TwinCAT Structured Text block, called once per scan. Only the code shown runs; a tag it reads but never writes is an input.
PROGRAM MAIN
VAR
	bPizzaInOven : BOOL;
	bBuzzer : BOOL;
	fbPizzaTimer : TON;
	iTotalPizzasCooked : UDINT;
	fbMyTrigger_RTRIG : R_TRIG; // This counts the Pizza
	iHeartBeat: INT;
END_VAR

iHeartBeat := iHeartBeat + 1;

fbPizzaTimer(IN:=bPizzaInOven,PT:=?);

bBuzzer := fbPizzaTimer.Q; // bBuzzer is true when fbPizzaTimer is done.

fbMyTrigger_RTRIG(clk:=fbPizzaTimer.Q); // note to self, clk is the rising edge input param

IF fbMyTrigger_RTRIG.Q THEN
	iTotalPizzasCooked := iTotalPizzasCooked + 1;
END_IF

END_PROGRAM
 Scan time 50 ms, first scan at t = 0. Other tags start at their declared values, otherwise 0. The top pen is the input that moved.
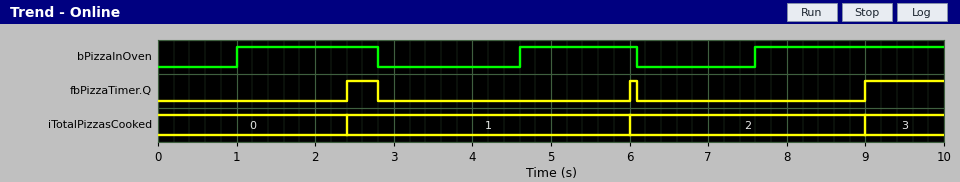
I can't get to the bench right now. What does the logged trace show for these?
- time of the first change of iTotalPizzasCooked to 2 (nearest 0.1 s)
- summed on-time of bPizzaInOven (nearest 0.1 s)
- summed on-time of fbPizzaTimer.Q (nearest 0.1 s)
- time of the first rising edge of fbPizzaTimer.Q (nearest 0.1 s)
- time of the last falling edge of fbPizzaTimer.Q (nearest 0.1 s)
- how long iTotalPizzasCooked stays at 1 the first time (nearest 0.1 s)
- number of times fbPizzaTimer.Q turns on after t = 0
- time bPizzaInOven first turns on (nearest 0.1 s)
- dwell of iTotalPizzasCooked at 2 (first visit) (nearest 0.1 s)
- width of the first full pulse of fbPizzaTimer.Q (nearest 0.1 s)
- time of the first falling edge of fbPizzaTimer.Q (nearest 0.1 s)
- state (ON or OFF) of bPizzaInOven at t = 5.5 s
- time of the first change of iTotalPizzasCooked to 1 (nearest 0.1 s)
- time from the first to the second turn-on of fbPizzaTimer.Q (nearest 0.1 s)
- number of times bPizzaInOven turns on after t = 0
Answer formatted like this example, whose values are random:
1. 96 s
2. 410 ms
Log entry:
1. 6.0 s
2. 5.7 s
3. 1.5 s
4. 2.4 s
5. 6.1 s
6. 3.6 s
7. 3
8. 1.0 s
9. 3.0 s
10. 0.4 s
11. 2.8 s
12. ON
13. 2.4 s
14. 3.6 s
15. 3
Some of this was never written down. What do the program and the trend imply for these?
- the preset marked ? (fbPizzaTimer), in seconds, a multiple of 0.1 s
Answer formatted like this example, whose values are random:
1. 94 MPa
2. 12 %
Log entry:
1. 1.4 s
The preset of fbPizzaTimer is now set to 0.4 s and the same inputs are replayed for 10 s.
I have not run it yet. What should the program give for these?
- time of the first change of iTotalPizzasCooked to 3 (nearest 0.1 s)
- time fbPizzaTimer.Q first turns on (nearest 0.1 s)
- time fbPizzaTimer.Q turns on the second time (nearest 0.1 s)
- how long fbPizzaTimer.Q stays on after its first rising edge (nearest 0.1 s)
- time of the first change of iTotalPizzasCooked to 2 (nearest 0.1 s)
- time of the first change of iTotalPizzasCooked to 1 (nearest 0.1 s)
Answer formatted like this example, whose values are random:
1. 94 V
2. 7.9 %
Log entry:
1. 8.0 s
2. 1.4 s
3. 5.0 s
4. 1.4 s
5. 5.0 s
6. 1.4 s
